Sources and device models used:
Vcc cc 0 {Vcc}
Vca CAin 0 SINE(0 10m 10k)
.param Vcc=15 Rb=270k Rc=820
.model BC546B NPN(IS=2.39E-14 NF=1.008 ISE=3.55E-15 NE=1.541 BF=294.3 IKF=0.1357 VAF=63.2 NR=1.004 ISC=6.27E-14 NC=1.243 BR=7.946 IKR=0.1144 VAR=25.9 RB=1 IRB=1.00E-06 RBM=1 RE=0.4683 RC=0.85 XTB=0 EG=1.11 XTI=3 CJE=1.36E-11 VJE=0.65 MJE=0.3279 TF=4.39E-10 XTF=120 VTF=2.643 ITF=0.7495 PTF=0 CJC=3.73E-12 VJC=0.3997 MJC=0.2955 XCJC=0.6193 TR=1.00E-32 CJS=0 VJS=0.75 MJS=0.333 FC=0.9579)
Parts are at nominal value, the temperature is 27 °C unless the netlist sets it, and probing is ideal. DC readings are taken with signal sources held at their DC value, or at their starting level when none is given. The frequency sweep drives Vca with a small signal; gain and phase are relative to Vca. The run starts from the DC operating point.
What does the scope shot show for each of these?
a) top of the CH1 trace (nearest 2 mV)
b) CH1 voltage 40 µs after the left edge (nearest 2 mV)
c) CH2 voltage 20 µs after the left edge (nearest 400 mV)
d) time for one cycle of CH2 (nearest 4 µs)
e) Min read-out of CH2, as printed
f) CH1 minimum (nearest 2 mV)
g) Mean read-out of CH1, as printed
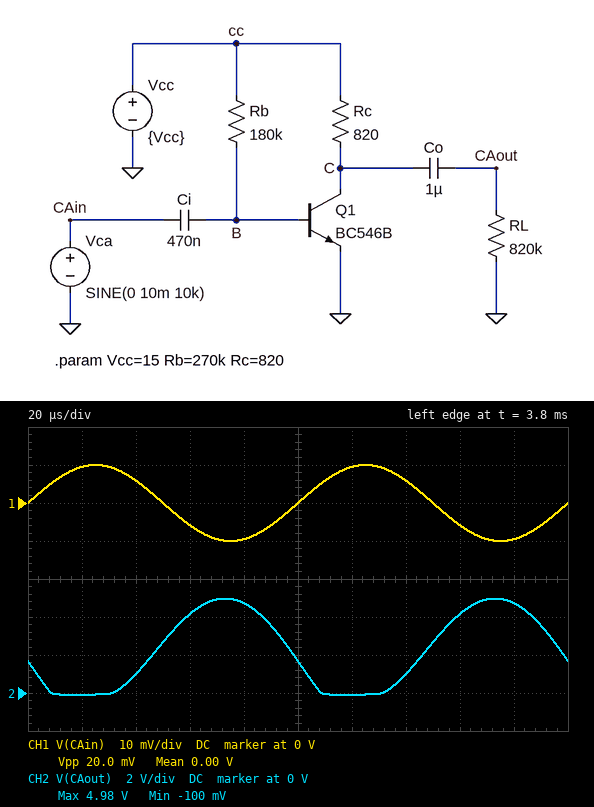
10 mV
6 mV
0 V
100 µs
-100 mV
-10 mV
0.00 V
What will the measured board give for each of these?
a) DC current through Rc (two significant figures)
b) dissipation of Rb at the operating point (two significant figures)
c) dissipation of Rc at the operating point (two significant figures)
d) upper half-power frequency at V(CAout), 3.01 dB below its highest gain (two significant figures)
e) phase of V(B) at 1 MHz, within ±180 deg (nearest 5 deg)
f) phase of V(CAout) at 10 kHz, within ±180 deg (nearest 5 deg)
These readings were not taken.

18 mA
1.1 mW
270 mW
9.5 MHz
0 deg
-125 deg
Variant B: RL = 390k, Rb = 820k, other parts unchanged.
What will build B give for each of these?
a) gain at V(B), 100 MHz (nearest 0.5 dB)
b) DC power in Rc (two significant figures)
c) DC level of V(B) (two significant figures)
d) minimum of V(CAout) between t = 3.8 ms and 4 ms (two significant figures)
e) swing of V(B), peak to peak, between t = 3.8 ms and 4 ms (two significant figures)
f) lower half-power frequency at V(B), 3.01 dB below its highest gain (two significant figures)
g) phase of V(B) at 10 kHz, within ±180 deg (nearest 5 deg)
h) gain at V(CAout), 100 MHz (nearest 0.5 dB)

0 dB
25 mW
680 mV
-1.5 V
20 mV
210 Hz
0 deg
41.0 dB
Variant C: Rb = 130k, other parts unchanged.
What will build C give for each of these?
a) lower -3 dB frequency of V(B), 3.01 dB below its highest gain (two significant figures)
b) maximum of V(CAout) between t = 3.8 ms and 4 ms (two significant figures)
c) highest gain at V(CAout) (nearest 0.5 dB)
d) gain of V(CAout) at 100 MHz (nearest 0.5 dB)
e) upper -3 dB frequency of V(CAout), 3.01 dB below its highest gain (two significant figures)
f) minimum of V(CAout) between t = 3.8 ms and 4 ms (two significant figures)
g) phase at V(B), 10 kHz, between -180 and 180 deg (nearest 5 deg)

23 kHz
4.3 V
33.5 dB
21.5 dB
26 MHz
-56 mV
65 deg
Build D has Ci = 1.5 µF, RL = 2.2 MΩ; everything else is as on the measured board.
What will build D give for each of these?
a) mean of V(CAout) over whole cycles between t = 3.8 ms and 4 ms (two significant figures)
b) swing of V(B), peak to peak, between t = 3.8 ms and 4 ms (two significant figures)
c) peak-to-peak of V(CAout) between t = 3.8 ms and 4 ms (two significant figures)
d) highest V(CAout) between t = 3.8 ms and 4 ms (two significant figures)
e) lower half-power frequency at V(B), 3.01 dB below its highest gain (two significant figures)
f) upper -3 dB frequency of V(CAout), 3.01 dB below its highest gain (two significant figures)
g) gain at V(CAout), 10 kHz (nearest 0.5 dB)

2.4 V
20 mV
5.3 V
5.2 V
4.4 kHz
9.4 MHz
43.5 dB
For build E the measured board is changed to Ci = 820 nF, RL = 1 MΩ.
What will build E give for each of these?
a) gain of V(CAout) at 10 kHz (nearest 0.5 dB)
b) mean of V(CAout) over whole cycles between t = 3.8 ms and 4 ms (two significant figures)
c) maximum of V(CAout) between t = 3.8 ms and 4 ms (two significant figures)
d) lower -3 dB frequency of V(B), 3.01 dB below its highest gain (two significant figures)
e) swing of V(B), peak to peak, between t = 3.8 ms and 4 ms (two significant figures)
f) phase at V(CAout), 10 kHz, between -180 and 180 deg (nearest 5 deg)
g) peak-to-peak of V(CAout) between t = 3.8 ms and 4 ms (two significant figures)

42.0 dB
2.4 V
5.1 V
8.1 kHz
20 mV
-140 deg
5.2 V
